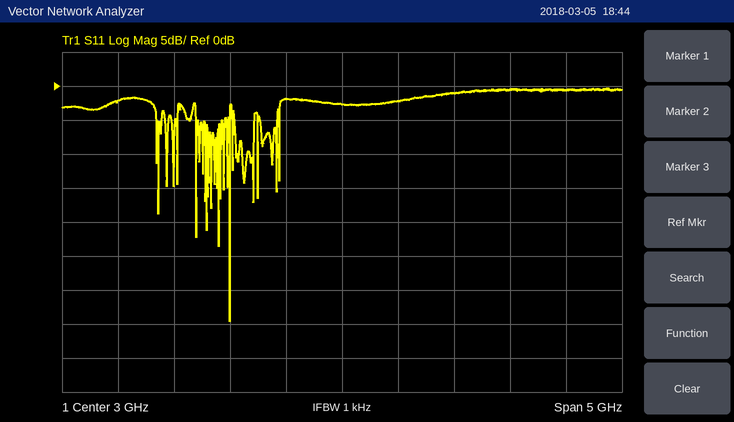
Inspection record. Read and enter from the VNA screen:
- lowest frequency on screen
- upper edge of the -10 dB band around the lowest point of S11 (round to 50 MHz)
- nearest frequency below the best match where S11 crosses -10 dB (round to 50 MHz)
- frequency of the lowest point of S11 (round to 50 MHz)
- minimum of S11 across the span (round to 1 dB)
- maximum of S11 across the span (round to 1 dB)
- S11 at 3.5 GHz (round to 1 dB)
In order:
500 MHz
2.00 GHz
2.00 GHz
2.00 GHz
-35 dB
0 dB
-2 dB
